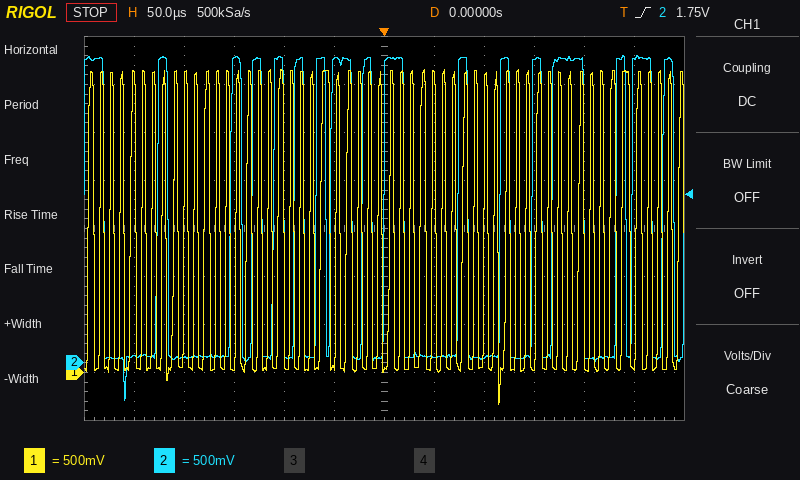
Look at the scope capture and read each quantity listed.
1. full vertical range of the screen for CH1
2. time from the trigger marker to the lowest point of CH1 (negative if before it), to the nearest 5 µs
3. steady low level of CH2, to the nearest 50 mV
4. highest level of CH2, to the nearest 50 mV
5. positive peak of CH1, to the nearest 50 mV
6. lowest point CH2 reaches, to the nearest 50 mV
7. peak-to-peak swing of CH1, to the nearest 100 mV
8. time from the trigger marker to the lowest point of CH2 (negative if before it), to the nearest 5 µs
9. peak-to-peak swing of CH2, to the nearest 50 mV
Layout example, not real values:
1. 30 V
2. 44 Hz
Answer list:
1. 4 V
2. +115 µs
3. 50 mV
4. 3.20 V
5. 3.15 V
6. -400 mV
7. 3.50 V
8. -260 µs
9. 3.60 V
